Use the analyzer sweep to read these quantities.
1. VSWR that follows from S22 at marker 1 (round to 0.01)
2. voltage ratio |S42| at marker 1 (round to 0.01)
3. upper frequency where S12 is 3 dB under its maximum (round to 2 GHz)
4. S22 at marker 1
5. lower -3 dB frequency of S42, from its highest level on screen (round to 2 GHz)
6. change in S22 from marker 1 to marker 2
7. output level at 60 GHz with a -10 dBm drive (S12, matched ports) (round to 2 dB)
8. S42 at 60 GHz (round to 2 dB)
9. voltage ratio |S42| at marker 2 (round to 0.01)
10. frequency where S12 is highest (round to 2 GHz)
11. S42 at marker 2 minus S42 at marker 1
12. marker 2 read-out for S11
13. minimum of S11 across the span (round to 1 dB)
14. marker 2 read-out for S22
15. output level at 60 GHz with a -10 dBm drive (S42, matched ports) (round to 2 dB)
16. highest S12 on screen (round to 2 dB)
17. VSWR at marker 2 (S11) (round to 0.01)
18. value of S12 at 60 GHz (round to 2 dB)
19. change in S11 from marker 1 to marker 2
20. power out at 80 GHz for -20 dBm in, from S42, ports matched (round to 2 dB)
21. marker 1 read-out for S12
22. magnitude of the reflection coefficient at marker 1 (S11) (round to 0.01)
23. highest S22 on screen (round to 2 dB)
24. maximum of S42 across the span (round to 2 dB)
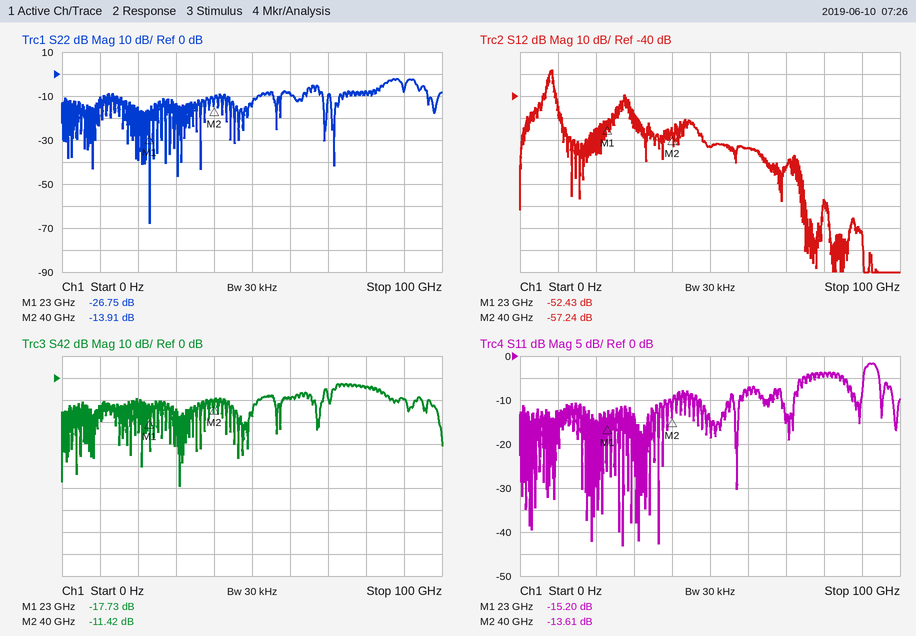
1.10
0.13
8 GHz
-26.75 dB
72 GHz
12.84 dB
-74 dBm
-10 dB
0.27
8 GHz
6.31 dB
-13.61 dB
-43 dB
-13.91 dB
-20 dBm
-28 dB
1.53
-64 dB
1.59 dB
-24 dBm
-52.43 dB
0.17
-2 dB
-2 dB
